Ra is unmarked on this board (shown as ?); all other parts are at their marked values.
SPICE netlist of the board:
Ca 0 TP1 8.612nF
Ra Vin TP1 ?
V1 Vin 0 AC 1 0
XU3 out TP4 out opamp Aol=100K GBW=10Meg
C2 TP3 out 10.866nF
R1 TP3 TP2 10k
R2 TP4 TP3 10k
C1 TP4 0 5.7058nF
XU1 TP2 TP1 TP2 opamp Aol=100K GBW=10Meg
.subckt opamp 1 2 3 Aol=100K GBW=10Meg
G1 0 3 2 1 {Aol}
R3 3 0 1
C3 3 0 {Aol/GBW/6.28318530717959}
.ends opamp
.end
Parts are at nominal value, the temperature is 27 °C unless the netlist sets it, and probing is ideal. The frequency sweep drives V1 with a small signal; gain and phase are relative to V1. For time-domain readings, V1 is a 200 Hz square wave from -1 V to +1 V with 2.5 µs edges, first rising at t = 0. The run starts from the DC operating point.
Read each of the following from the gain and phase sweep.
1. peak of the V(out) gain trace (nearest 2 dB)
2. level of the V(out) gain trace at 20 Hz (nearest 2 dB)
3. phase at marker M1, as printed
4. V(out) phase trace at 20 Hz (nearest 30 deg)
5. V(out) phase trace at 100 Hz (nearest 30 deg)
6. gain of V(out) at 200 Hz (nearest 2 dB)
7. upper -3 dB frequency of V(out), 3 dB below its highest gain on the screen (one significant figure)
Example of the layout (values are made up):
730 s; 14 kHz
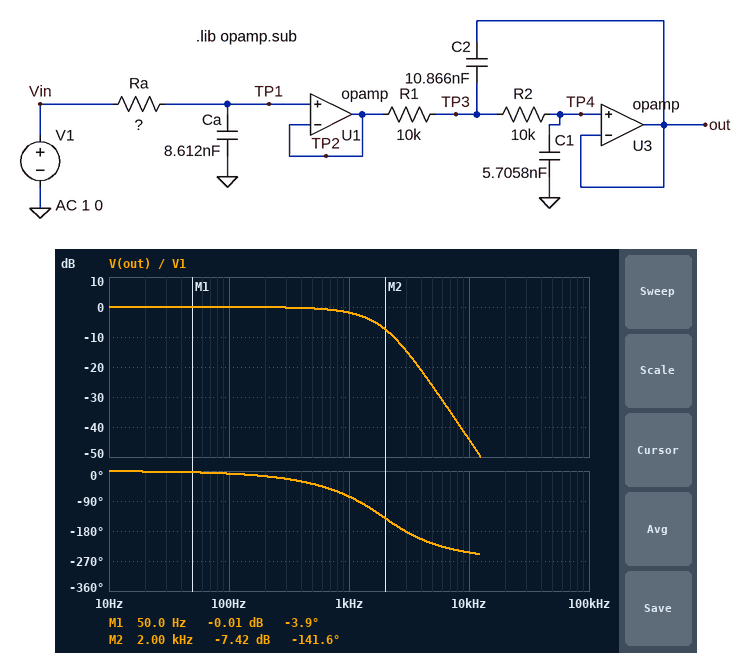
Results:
0 dB; 0 dB; -3.9 deg; 0 deg; 0 deg; 0 dB; 1 kHz
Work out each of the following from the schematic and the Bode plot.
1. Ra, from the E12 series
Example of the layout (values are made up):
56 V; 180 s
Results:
12 kΩ
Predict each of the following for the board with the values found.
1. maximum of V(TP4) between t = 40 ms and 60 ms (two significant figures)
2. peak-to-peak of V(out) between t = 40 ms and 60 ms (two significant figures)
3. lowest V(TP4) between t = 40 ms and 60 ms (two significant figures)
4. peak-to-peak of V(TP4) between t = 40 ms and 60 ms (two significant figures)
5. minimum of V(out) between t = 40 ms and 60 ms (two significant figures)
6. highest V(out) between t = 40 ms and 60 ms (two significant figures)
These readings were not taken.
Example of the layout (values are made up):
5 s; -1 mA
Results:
1.0 V; 2.0 V; -1.0 V; 2.0 V; -1.0 V; 1.0 V
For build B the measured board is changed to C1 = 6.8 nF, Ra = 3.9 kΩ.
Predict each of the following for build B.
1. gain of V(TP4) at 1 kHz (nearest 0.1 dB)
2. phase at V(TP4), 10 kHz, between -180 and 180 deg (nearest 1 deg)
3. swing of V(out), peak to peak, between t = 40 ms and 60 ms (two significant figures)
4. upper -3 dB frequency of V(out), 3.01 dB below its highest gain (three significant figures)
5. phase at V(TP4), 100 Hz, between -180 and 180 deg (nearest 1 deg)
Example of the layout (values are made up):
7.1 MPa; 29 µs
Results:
-1.1 dB; 132 deg; 2.1 V; 1.53 kHz; -6 deg
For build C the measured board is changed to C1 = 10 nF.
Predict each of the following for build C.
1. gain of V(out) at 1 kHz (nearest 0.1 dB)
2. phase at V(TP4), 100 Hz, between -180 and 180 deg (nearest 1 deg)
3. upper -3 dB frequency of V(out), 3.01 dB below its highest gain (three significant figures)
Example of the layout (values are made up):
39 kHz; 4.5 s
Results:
-4.3 dB; -11 deg; 816 Hz
